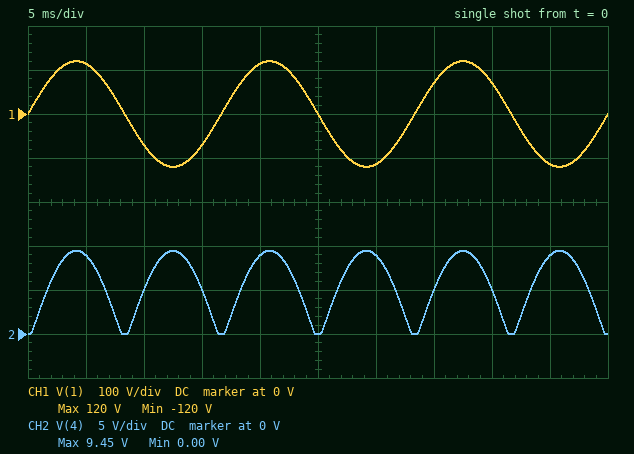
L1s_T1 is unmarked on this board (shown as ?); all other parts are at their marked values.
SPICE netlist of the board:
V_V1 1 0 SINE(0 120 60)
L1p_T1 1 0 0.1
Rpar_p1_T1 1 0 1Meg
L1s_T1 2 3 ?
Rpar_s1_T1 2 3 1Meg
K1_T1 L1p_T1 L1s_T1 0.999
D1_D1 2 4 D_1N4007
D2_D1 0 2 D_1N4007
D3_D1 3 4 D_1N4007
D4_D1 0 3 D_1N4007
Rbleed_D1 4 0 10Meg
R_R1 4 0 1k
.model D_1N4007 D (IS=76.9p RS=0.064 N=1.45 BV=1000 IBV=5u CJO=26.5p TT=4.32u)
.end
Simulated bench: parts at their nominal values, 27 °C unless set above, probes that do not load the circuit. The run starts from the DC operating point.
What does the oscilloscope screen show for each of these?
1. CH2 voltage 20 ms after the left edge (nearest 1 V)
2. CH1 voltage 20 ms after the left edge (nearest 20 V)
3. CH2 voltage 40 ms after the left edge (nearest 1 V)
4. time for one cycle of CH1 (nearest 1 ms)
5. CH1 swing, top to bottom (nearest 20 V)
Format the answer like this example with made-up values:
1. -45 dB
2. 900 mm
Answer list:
1. 9 V
2. 120 V
3. 5 V
4. 17 ms
5. 240 V
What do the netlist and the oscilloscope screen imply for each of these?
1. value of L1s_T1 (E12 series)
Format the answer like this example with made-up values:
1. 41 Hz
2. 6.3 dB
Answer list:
1. 820 µH
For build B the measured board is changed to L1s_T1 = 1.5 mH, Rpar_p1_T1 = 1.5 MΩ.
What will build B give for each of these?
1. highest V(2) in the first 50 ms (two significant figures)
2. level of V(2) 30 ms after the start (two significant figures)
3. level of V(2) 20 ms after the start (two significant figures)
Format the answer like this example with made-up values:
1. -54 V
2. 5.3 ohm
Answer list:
1. 14 V
2. -710 mV
3. 13 V
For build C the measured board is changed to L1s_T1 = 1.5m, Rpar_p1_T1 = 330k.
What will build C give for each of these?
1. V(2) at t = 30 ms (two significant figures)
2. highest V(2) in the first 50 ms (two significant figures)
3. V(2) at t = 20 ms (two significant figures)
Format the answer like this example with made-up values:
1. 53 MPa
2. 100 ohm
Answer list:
1. -710 mV
2. 14 V
3. 13 V
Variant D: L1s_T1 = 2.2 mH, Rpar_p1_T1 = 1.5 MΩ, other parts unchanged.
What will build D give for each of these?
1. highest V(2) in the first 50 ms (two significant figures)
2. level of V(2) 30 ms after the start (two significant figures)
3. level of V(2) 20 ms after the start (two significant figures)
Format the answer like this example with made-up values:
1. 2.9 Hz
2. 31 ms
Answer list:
1. 17 V
2. -720 mV
3. 16 V
